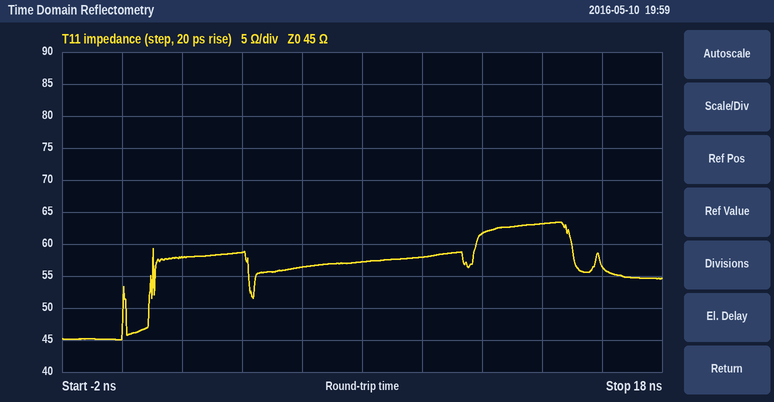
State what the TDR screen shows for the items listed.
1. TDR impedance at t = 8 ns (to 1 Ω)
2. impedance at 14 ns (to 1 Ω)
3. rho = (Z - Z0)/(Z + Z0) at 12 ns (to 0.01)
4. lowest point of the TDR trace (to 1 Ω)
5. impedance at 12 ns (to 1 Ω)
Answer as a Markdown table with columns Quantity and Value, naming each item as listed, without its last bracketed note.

| Quantity | Value |
|---|---|
| TDR impedance at t = 8 ns | 57 Ω |
| impedance at 14 ns | 63 Ω |
| rho = (Z - Z0)/(Z + Z0) at 12 ns | +0.16 |
| lowest point of the TDR trace | 45 Ω |
| impedance at 12 ns | 62 Ω |
